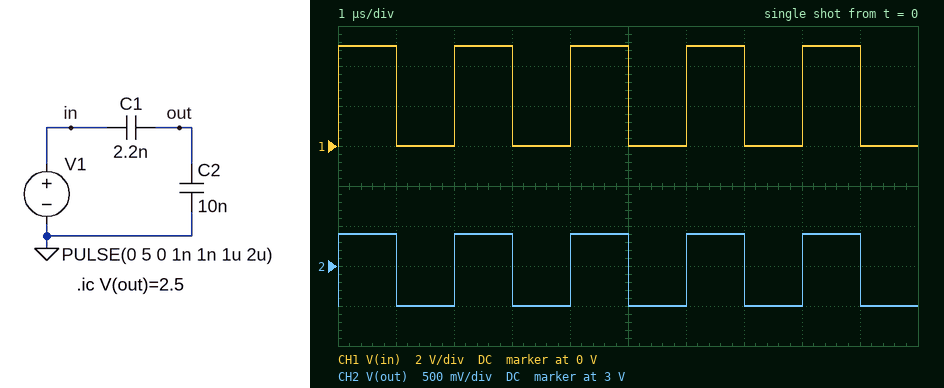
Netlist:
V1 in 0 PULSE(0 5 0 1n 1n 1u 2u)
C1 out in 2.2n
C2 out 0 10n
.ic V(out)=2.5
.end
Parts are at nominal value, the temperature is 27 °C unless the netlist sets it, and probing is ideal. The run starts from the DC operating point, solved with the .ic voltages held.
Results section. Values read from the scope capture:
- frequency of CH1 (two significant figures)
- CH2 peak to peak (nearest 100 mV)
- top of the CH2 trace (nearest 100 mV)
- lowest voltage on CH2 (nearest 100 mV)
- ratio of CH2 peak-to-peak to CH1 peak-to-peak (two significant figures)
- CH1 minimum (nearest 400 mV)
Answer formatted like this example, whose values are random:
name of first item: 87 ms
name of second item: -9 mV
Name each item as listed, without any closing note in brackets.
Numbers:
frequency of CH1: 500 kHz
CH2 peak to peak: 900 mV
top of the CH2 trace: 3.4 V
lowest voltage on CH2: 2.5 V
ratio of CH2 peak-to-peak to CH1 peak-to-peak: 0.18
CH1 minimum: 0 V
